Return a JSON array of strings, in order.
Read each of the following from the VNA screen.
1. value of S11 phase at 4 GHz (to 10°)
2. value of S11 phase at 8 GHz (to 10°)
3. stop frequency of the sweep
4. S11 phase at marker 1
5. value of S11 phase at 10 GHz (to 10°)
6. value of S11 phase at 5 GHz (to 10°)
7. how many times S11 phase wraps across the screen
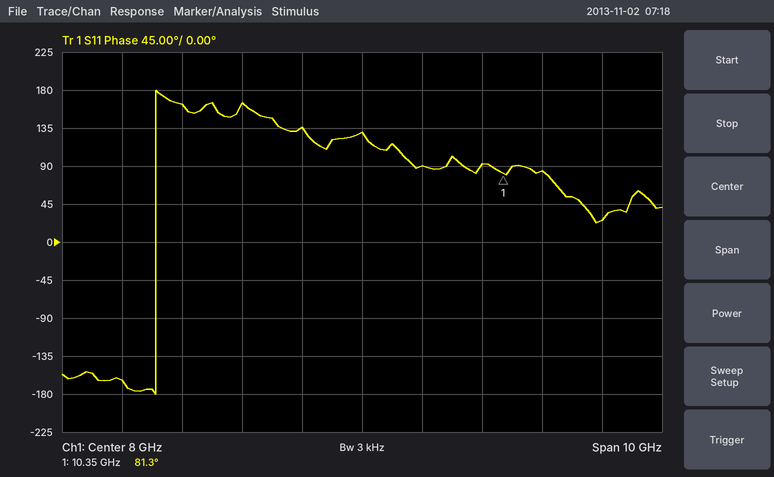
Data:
["-160°", "130°", "13 GHz", "81.3°", "90°", "160°", "1"]
